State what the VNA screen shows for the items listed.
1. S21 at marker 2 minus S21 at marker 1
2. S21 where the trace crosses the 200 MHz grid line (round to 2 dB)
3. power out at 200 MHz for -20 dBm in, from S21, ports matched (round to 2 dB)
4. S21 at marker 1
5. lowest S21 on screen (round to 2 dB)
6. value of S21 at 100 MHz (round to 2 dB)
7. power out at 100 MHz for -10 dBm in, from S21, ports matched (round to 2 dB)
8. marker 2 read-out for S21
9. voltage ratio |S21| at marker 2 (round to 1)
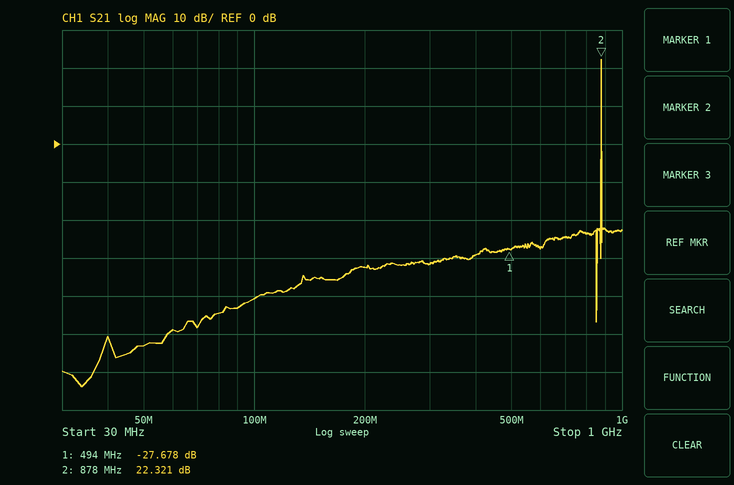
49.999 dB
-32 dB
-52 dBm
-27.678 dB
-64 dB
-40 dB
-50 dBm
22.321 dB
13
